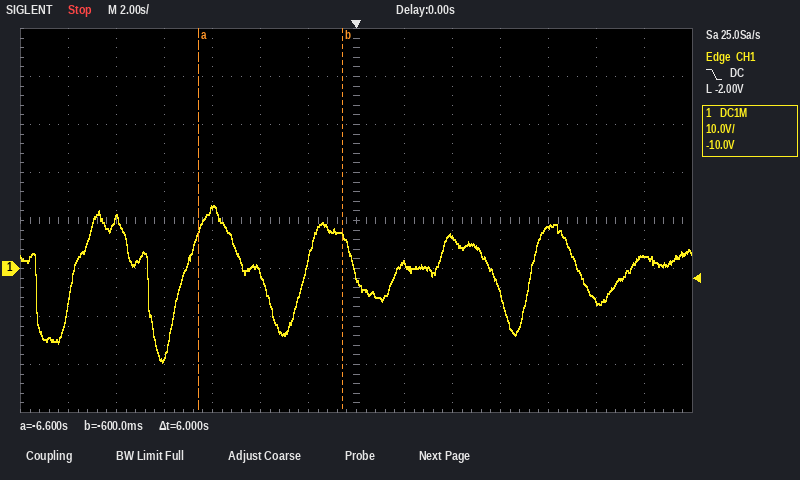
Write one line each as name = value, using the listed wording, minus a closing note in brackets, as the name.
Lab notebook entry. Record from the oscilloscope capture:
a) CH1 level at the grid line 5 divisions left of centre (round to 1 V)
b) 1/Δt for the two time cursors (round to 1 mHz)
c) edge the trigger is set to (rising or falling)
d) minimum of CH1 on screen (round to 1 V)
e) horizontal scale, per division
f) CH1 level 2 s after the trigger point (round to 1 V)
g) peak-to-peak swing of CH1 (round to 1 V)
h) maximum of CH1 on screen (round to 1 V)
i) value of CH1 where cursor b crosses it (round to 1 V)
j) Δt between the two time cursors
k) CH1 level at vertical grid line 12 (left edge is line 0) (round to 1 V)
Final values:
CH1 level at the grid line 5 divisions left of centre = 10 V
1/Δt for the two time cursors = 167 mHz
edge the trigger is set to = falling
minimum of CH1 on screen = -20 V
horizontal scale, per division = 2 s
CH1 level 2 s after the trigger point = 1 V
peak-to-peak swing of CH1 = 33 V
maximum of CH1 on screen = 13 V
value of CH1 where cursor b crosses it = 7 V
Δt between the two time cursors = 6 s
CH1 level at vertical grid line 12 (left edge is line 0) = -7 V
